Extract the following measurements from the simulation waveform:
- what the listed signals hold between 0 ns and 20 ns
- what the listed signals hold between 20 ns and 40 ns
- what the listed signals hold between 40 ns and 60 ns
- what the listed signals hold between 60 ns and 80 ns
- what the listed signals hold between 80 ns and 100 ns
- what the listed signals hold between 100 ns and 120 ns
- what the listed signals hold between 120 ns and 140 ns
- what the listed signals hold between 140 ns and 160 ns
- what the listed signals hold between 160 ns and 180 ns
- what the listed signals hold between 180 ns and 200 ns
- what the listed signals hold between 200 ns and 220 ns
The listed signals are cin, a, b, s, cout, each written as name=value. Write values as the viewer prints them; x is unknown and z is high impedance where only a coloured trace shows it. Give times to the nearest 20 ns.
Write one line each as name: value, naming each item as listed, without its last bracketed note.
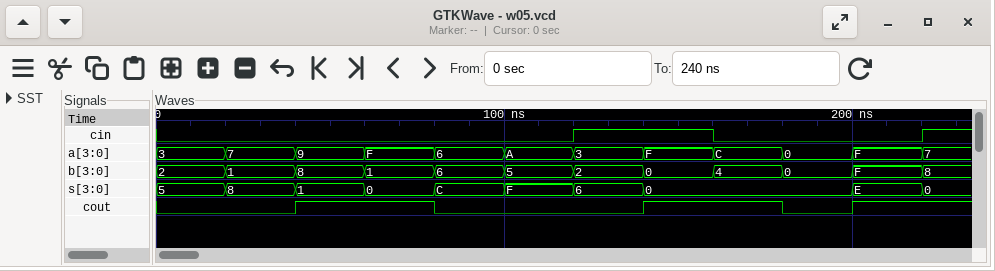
what the listed signals hold between 0 ns and 20 ns: cin=0, a=3, b=2, s=5, cout=0
what the listed signals hold between 20 ns and 40 ns: cin=0, a=7, b=1, s=8, cout=0
what the listed signals hold between 40 ns and 60 ns: cin=0, a=9, b=8, s=1, cout=1
what the listed signals hold between 60 ns and 80 ns: cin=0, a=F, b=1, s=0, cout=1
what the listed signals hold between 80 ns and 100 ns: cin=0, a=6, b=6, s=C, cout=0
what the listed signals hold between 100 ns and 120 ns: cin=0, a=A, b=5, s=F, cout=0
what the listed signals hold between 120 ns and 140 ns: cin=1, a=3, b=2, s=6, cout=0
what the listed signals hold between 140 ns and 160 ns: cin=1, a=F, b=0, s=0, cout=1
what the listed signals hold between 160 ns and 180 ns: cin=0, a=C, b=4, s=0, cout=1
what the listed signals hold between 180 ns and 200 ns: cin=0, a=0, b=0, s=0, cout=0
what the listed signals hold between 200 ns and 220 ns: cin=0, a=F, b=F, s=E, cout=1
